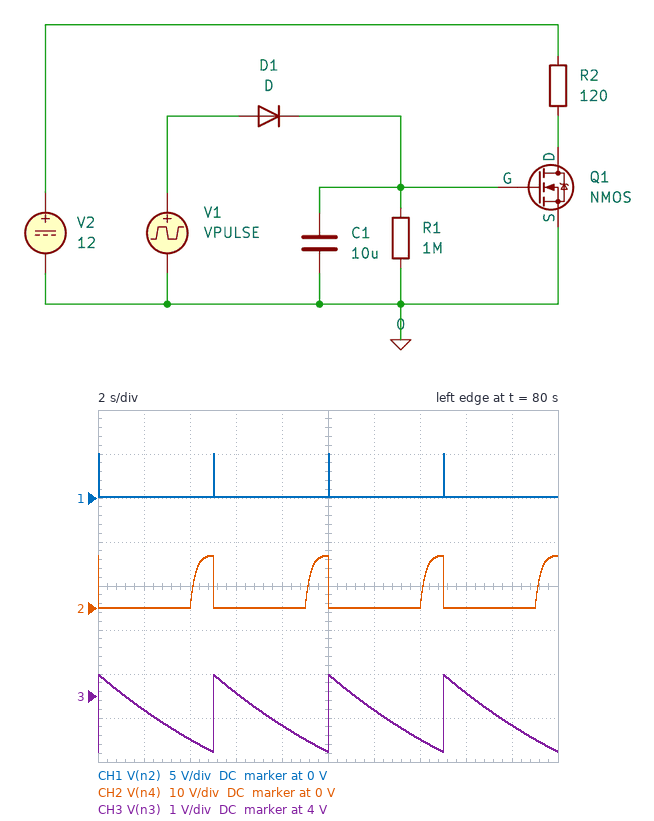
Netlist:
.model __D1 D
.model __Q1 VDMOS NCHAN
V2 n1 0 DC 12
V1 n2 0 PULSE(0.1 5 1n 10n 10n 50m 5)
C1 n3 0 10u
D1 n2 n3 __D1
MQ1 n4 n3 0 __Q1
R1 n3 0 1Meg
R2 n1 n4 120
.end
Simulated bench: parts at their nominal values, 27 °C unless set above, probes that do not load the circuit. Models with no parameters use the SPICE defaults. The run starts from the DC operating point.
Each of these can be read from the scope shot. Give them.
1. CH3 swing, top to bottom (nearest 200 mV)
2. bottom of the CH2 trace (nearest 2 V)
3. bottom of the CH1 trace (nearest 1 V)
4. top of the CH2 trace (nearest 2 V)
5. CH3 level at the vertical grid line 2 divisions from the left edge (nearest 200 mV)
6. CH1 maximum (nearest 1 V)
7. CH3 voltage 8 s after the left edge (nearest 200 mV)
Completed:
1.8 V
0 V
0 V
12 V
3.0 V
5 V
3.4 V
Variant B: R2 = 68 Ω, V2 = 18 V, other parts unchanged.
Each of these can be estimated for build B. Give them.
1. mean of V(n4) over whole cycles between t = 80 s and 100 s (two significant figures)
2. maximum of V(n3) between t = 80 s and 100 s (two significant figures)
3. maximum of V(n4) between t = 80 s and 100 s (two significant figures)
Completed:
3.6 V
4.5 V
18 V
